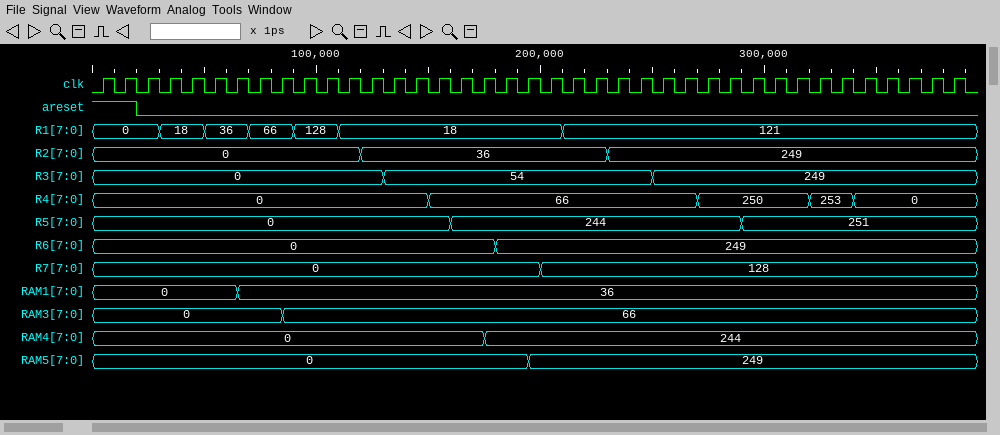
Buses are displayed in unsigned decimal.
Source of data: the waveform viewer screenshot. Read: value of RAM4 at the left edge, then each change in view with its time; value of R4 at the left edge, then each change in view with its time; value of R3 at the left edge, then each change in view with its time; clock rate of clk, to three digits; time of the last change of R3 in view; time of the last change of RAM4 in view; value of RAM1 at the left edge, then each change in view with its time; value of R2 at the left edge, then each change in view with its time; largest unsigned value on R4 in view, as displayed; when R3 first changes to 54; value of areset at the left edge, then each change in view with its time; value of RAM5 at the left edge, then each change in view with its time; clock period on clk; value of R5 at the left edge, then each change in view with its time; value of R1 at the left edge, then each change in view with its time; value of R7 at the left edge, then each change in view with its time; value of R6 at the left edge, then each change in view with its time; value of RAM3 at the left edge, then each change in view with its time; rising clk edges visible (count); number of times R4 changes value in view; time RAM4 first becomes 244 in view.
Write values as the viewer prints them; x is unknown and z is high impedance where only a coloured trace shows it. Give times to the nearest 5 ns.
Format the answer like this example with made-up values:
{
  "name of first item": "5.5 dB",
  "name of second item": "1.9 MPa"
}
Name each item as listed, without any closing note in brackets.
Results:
{
  "value of RAM4 at the left edge, then each change in view with its time": "0, 244 at 175 ns",
  "value of R4 at the left edge, then each change in view with its time": "0, 66 at 150 ns, 250 at 270 ns, 253 at 320 ns, 0 at 340 ns",
  "value of R3 at the left edge, then each change in view with its time": "0, 54 at 130 ns, 249 at 250 ns",
  "clock rate of clk, to three digits": "100 MHz",
  "time of the last change of R3 in view": "250 ns",
  "time of the last change of RAM4 in view": "175 ns",
  "value of RAM1 at the left edge, then each change in view with its time": "0, 36 at 65 ns",
  "value of R2 at the left edge, then each change in view with its time": "0, 36 at 120 ns, 249 at 230 ns",
  "largest unsigned value on R4 in view, as displayed": "253",
  "when R3 first changes to 54": "130 ns",
  "value of areset at the left edge, then each change in view with its time": "1, 0 at 20 ns",
  "value of RAM5 at the left edge, then each change in view with its time": "0, 249 at 195 ns",
  "clock period on clk": "10 ns",
  "value of R5 at the left edge, then each change in view with its time": "0, 244 at 160 ns, 251 at 290 ns",
  "value of R1 at the left edge, then each change in view with its time": "0, 18 at 30 ns, 36 at 50 ns, 66 at 70 ns, 128 at 90 ns, 18 at 110 ns, 121 at 210 ns",
  "value of R7 at the left edge, then each change in view with its time": "0, 128 at 200 ns",
  "value of R6 at the left edge, then each change in view with its time": "0, 249 at 180 ns",
  "value of RAM3 at the left edge, then each change in view with its time": "0, 66 at 85 ns",
  "rising clk edges visible": "39",
  "number of times R4 changes value in view": "4",
  "time RAM4 first becomes 244 in view": "175 ns"
}
